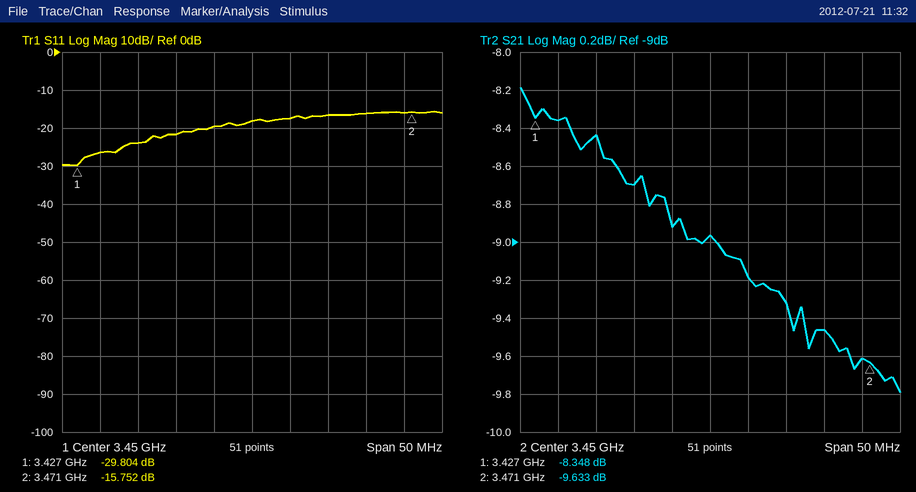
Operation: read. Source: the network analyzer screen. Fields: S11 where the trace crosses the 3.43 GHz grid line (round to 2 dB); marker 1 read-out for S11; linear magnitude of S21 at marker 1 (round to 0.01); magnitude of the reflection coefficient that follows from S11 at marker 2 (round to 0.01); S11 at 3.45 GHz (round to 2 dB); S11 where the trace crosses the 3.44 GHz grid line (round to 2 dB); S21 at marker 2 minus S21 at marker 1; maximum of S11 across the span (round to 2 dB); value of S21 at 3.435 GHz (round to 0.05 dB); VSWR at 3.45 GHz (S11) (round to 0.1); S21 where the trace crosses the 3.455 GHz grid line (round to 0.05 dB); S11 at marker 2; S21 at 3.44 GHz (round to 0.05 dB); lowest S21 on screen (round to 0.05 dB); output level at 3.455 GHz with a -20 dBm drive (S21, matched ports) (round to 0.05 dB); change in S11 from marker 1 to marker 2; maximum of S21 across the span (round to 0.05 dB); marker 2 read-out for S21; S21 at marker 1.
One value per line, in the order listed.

-26 dB
-29.804 dB
0.38
0.16
-18 dB
-22 dB
-1.285 dB
-16 dB
-8.45 dB
1.3
-9.20 dB
-15.752 dB
-8.70 dB
-9.80 dB
-29.20 dBm
14.052 dB
-8.20 dB
-9.633 dB
-8.348 dB
